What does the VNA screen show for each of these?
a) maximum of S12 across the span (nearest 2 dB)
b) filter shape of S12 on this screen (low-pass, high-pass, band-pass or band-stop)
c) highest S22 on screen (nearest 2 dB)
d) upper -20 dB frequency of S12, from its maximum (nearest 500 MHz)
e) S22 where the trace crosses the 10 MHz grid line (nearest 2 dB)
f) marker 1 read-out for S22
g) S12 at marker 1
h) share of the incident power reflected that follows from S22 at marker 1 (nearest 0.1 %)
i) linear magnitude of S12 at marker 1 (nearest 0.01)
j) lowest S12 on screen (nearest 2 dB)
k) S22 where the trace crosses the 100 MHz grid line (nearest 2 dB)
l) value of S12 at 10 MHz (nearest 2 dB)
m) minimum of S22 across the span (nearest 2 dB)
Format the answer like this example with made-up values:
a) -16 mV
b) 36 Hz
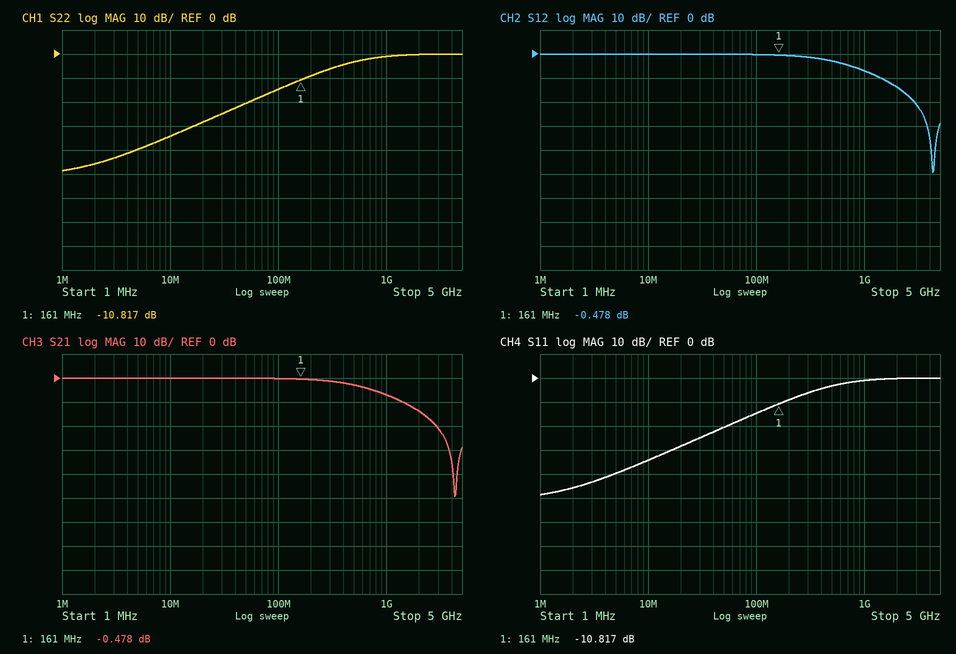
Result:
a) 0 dB
b) low-pass
c) 0 dB
d) 3.0 GHz
e) -34 dB
f) -10.817 dB
g) -0.478 dB
h) 8.3 %
i) 0.95
j) -50 dB
k) -14 dB
l) 0 dB
m) -48 dB
